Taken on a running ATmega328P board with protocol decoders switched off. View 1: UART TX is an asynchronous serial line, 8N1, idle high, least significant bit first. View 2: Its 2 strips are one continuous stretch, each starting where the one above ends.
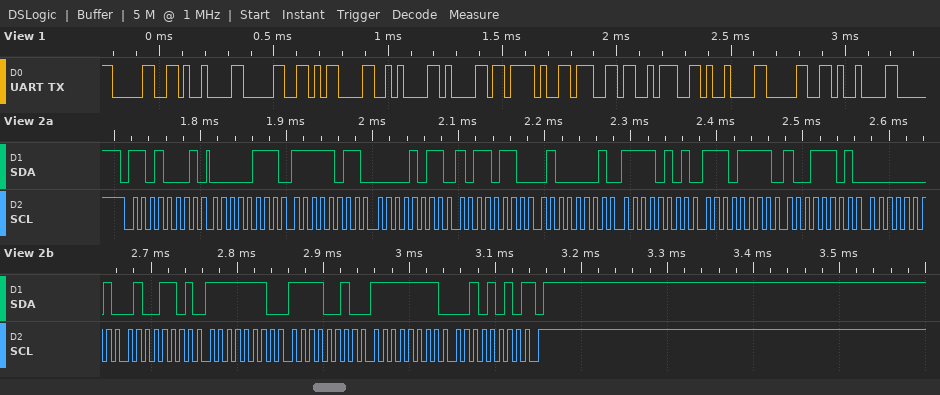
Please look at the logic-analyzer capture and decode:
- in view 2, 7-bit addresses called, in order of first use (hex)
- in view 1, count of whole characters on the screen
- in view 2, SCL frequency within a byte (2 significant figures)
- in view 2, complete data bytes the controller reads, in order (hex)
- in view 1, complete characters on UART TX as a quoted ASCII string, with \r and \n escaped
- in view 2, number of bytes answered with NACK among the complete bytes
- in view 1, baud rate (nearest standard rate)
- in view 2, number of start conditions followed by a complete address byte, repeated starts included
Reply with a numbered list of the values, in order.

1. 0x68
2. 12
3. 100 kHz
4. 07 FB 0B B6 41 F5 EF 9D 01 4D FE F2 FF 2A
5. "0\t0\r\na/g:\t0\t"
6. 1
7. 38400 baud
8. 1
